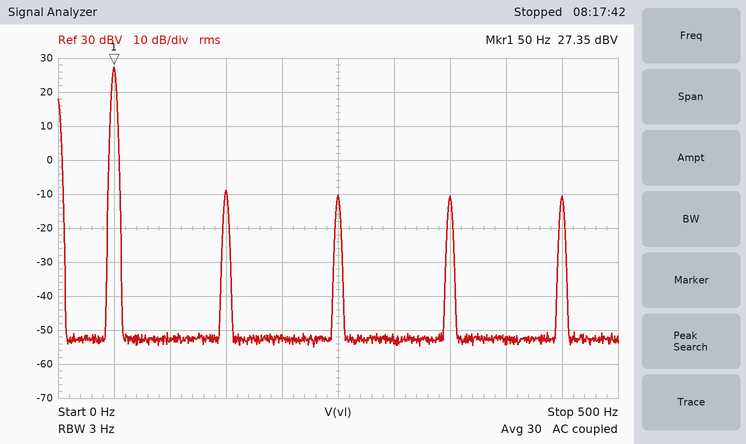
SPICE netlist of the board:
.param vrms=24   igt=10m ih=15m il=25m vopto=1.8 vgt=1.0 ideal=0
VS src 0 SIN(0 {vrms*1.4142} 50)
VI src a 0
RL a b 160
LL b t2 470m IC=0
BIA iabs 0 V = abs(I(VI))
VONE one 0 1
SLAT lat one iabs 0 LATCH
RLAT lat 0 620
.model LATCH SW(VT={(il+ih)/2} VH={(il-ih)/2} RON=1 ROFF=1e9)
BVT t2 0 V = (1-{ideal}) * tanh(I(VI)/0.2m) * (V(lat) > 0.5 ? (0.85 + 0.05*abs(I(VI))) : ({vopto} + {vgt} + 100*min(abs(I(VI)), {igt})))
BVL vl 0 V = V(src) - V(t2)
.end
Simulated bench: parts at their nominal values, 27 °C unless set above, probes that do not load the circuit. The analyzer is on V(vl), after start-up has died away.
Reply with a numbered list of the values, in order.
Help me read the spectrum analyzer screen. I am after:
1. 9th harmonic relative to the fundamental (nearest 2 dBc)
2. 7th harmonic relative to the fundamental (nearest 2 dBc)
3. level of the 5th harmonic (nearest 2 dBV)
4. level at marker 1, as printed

1. -38 dBc
2. -38 dBc
3. -10 dBV
4. 27.35 dBV
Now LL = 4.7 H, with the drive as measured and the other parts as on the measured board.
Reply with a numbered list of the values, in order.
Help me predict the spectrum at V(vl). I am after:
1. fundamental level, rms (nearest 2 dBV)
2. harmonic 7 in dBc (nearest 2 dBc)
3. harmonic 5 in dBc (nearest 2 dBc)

1. 28 dBV
2. -36 dBc
3. -32 dBc
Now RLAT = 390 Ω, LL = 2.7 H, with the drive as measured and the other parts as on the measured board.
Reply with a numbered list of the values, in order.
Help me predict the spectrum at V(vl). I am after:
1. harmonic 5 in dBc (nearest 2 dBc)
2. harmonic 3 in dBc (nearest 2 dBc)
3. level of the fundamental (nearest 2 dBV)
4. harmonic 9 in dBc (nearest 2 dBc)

1. -28 dBc
2. -26 dBc
3. 28 dBV
4. -36 dBc
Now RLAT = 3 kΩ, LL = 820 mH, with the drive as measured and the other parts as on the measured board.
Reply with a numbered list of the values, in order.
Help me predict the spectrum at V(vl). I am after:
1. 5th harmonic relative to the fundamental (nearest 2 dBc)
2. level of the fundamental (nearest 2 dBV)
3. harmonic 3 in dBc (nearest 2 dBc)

1. -36 dBc
2. 28 dBV
3. -34 dBc
